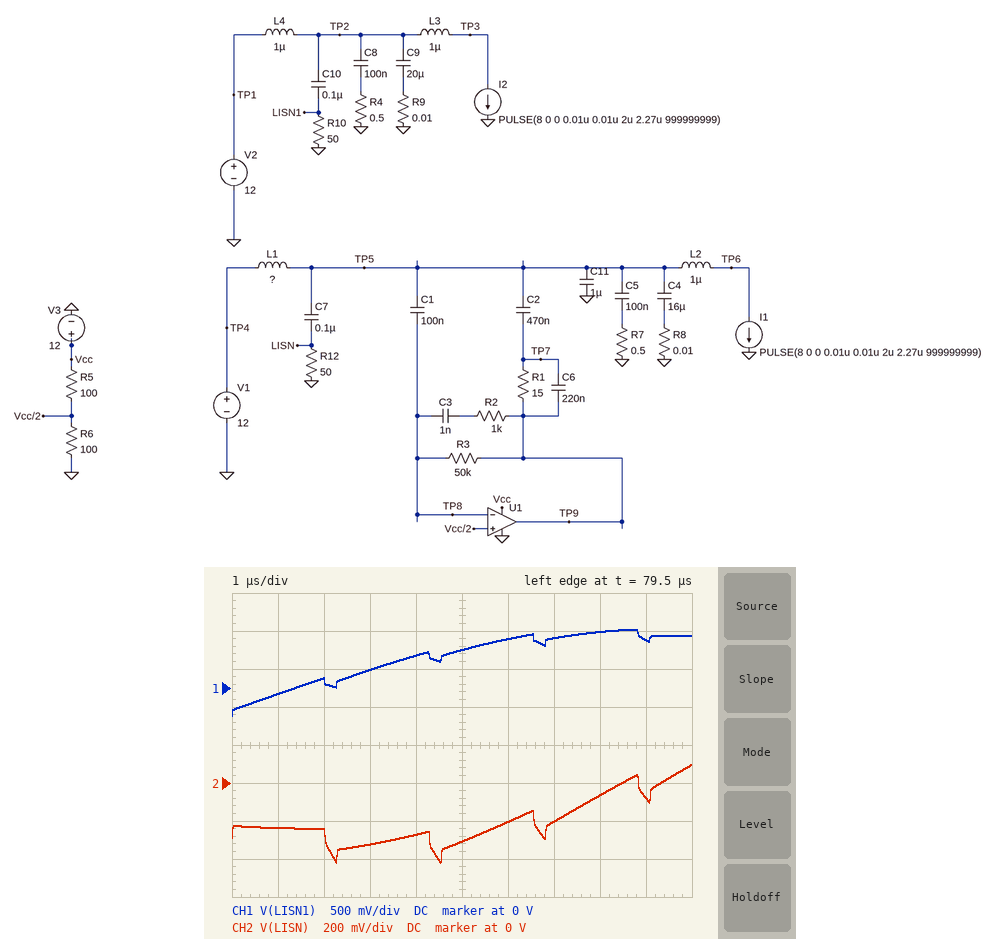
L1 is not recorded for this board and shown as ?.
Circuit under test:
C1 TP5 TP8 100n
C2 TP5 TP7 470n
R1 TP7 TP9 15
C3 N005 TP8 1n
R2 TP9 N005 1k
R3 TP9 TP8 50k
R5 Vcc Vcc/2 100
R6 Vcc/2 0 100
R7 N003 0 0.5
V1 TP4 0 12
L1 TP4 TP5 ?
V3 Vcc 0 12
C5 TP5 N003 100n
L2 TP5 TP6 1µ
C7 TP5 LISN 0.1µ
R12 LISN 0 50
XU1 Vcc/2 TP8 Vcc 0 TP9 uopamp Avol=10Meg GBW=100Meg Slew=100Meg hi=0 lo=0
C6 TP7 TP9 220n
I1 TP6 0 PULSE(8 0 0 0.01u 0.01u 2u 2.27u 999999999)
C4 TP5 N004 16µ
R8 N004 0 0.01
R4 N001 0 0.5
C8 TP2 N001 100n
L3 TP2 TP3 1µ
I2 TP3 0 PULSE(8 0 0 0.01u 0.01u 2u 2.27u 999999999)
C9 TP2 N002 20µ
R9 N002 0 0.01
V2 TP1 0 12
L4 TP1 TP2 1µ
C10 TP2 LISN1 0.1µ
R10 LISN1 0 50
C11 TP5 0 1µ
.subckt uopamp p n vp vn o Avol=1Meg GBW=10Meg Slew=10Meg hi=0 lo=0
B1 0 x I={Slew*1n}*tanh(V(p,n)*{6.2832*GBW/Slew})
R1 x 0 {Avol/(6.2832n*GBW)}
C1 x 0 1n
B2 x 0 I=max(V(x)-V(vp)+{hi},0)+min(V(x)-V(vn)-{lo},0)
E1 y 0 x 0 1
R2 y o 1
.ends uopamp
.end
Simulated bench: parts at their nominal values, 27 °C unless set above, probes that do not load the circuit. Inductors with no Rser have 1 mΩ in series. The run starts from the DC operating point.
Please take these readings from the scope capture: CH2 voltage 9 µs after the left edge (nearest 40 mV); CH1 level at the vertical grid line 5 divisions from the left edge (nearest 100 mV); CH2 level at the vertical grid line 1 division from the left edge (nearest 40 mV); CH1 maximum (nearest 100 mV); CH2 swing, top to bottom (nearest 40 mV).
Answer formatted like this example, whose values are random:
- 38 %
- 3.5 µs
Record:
- -80 mV
- 500 mV
- -240 mV
- 800 mV
- 520 mV
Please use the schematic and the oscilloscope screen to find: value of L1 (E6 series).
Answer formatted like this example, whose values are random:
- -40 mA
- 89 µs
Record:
- 680 nH
